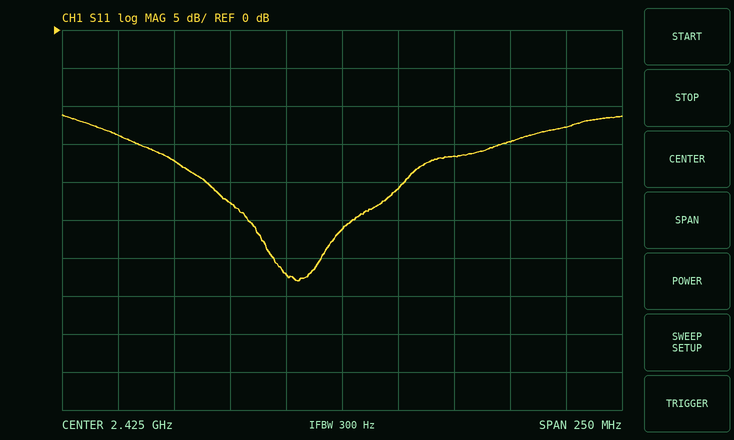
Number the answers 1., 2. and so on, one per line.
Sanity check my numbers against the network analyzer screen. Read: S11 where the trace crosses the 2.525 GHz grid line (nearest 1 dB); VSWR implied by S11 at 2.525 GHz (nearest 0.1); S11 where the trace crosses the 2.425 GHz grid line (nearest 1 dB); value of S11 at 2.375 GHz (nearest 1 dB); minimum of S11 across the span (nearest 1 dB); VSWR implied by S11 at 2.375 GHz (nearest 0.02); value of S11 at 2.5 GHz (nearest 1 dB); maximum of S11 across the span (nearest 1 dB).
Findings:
1. -13 dB
2. 1.6
3. -26 dB
4. -23 dB
5. -33 dB
6. 1.16
7. -15 dB
8. -11 dB
